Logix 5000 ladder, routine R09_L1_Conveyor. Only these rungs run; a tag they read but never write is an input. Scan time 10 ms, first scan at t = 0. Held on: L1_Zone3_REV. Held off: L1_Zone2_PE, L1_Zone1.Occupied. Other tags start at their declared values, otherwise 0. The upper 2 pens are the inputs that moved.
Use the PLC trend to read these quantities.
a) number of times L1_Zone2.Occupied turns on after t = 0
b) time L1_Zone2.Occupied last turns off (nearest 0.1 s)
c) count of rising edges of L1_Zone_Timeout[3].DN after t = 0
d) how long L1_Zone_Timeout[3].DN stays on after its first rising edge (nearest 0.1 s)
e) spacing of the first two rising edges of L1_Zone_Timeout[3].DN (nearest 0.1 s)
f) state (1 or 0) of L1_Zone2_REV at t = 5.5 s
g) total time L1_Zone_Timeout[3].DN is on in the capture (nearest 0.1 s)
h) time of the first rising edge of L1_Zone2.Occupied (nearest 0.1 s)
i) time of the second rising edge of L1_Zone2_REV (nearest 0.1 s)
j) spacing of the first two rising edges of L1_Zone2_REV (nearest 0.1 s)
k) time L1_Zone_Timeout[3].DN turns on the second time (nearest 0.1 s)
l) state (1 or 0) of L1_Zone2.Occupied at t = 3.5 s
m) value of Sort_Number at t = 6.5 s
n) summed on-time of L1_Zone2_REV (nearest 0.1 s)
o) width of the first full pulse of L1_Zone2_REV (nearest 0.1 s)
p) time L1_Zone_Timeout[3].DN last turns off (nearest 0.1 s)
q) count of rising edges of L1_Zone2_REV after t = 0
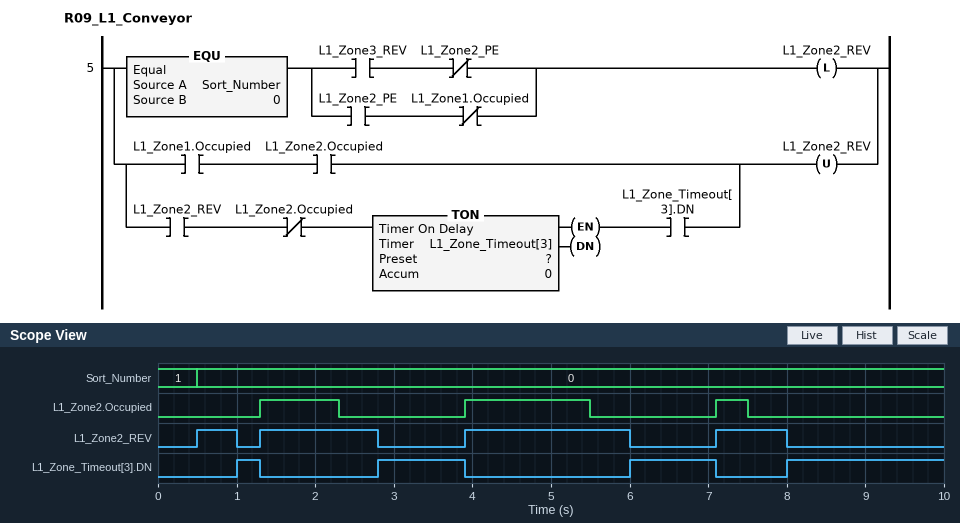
3
7.5 s
4
0.3 s
1.8 s
1
4.5 s
1.3 s
1.3 s
0.8 s
2.8 s
0
0
5.0 s
0.5 s
7.1 s
4
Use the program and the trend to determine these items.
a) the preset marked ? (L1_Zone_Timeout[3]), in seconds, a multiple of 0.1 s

0.5 s
